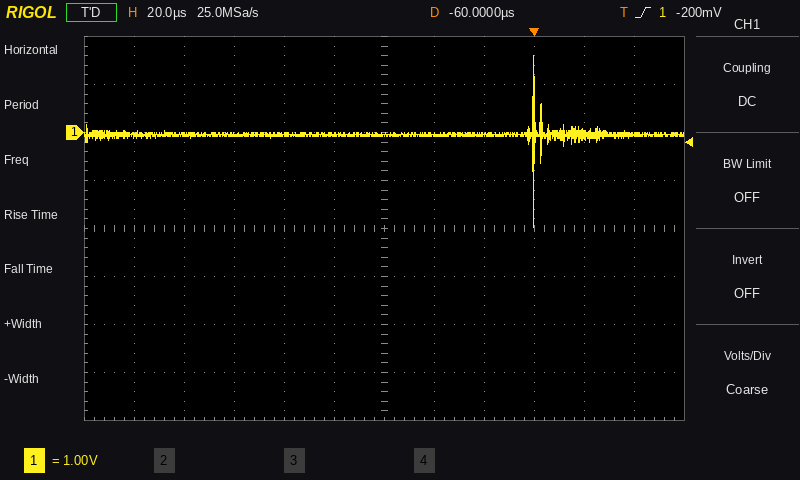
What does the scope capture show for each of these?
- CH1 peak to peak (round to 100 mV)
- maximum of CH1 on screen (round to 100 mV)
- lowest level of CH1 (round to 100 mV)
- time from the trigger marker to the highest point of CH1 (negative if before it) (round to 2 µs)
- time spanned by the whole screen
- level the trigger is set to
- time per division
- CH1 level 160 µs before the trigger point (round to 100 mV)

3.6 V
1.6 V
-2.0 V
0 µs
240 µs
-200 mV
20 µs
-100 mV
